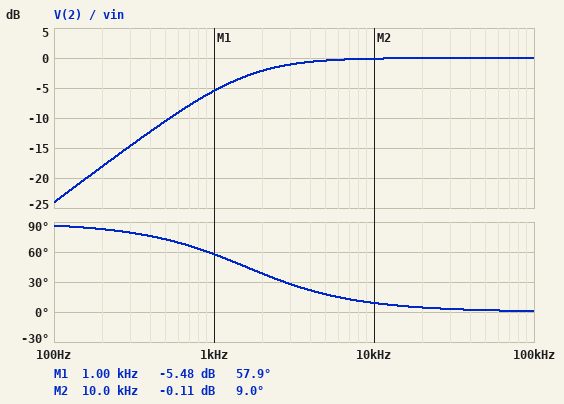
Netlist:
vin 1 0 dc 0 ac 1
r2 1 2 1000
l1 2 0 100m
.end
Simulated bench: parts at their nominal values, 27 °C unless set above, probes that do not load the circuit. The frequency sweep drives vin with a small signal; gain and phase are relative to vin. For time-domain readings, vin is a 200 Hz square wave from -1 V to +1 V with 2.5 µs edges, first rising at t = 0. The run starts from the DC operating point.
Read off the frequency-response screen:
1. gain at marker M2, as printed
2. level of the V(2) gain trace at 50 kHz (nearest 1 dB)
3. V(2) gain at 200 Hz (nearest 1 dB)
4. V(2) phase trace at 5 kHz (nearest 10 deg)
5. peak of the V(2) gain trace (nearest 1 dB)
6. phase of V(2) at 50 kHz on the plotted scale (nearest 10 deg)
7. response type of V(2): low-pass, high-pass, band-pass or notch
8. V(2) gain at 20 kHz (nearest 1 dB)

-0.11 dB
0 dB
-18 dB
20 deg
0 dB
0 deg
high-pass
0 dB
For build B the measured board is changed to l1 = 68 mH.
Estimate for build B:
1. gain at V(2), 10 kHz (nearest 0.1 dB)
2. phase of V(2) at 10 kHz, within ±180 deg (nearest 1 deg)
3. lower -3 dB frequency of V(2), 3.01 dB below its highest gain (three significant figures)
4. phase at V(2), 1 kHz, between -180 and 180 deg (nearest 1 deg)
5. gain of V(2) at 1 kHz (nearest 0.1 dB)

-0.2 dB
13 deg
2.34 kHz
67 deg
-8.1 dB
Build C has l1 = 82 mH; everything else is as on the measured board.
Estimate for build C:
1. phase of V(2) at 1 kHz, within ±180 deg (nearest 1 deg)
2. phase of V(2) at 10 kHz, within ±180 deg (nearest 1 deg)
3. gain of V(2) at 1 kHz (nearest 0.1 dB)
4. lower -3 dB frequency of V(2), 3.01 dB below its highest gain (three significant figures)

63 deg
11 deg
-6.8 dB
1.94 kHz
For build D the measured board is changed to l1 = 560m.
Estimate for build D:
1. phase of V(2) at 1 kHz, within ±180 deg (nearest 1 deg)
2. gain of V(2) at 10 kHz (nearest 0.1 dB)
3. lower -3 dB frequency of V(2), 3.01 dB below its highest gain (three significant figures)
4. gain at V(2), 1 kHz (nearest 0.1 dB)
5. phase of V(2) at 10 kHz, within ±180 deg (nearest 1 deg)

16 deg
0 dB
284 Hz
-0.3 dB
2 deg
